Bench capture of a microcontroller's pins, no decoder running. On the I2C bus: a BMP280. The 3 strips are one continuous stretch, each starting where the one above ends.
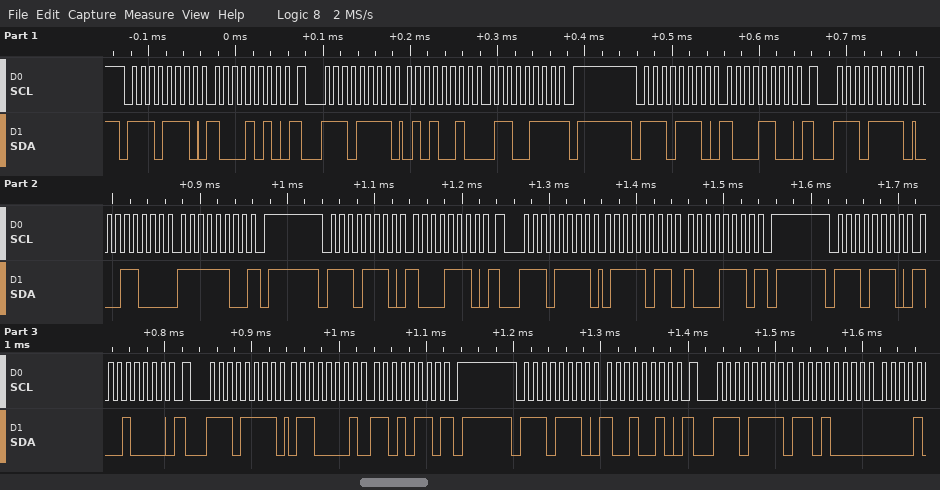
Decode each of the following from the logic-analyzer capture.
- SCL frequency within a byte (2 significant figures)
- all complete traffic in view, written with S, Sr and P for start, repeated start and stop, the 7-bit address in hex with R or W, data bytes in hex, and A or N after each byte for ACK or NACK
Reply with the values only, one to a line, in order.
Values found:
100 kHz
S 77W A 8A A Sr 77R A 52 A 67 N P S 77W A 8C A Sr 77R A 18 A FC N P S 77W A 8E A Sr 77R A 7B A 8E N P S 77W A 90 A Sr 77R A 61 A D6 N P S 77W A 92 A Sr 77R A D0 A
